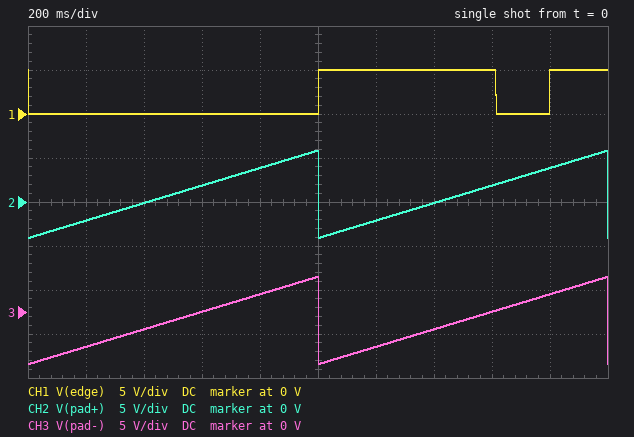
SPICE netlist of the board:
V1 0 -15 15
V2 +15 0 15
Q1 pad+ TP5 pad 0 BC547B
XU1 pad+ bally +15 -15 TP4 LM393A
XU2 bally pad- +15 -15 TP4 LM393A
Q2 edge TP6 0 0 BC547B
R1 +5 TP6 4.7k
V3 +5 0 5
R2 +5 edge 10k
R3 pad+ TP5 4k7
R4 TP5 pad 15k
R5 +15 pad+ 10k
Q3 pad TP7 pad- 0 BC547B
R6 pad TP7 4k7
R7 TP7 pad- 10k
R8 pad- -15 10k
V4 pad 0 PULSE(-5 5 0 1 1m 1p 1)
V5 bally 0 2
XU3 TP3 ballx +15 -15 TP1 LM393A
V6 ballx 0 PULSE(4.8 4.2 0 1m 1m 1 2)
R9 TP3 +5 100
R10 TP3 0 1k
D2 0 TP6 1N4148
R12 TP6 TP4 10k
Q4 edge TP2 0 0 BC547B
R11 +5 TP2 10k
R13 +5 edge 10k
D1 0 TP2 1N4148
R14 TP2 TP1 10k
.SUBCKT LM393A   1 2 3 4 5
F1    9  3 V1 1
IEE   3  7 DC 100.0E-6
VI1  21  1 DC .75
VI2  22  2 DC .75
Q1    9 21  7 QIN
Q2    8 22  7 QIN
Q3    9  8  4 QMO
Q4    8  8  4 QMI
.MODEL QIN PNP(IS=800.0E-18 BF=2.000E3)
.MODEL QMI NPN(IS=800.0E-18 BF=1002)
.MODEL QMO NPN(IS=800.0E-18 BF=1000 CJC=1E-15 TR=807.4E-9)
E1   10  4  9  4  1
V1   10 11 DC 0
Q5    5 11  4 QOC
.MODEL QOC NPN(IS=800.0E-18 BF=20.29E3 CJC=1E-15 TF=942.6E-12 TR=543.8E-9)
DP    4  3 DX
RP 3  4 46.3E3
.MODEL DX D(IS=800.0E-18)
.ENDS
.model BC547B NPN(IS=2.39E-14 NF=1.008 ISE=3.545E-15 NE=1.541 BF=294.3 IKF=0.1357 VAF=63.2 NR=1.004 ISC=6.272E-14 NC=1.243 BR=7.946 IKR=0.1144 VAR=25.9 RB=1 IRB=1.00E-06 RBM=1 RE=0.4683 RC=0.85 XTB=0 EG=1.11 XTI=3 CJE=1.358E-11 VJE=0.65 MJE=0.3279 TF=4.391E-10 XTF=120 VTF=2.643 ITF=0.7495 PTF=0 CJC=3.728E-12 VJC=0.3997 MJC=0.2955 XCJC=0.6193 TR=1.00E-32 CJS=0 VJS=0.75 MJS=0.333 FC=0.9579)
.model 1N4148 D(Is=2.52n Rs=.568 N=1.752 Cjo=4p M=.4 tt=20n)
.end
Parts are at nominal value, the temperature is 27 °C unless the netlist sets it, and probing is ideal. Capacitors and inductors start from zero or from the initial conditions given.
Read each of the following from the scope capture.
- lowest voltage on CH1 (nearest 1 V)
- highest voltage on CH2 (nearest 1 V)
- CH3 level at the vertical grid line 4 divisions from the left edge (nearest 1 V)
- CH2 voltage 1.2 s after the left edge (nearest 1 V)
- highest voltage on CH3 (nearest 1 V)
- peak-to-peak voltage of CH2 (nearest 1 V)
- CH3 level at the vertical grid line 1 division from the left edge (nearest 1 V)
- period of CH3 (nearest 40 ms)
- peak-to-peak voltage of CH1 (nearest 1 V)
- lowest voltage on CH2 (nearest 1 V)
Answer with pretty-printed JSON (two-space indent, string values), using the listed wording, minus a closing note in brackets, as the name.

{
  "lowest voltage on CH1": "0 V",
  "highest voltage on CH2": "6 V",
  "CH3 level at the vertical grid line 4 divisions from the left edge": "2 V",
  "CH2 voltage 1.2 s after the left edge": "-2 V",
  "highest voltage on CH3": "4 V",
  "peak-to-peak voltage of CH2": "10 V",
  "CH3 level at the vertical grid line 1 division from the left edge": "-4 V",
  "period of CH3": "1.00 s",
  "peak-to-peak voltage of CH1": "5 V",
  "lowest voltage on CH2": "-4 V"
}
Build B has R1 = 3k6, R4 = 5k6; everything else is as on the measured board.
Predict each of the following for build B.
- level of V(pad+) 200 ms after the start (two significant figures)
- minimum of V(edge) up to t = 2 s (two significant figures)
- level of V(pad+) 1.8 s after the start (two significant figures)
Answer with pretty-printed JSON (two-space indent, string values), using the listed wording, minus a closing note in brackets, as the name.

{
  "level of V(pad+) 200 ms after the start": "-1.8 V",
  "minimum of V(edge) up to t = 2 s": "10 mV",
  "level of V(pad+) 1.8 s after the start": "4.2 V"
}
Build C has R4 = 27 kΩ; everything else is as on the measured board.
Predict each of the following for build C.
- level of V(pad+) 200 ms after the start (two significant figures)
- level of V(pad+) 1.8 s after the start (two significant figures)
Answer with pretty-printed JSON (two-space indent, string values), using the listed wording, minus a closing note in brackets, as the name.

{
  "level of V(pad+) 200 ms after the start": "-2.2 V",
  "level of V(pad+) 1.8 s after the start": "3.8 V"
}
